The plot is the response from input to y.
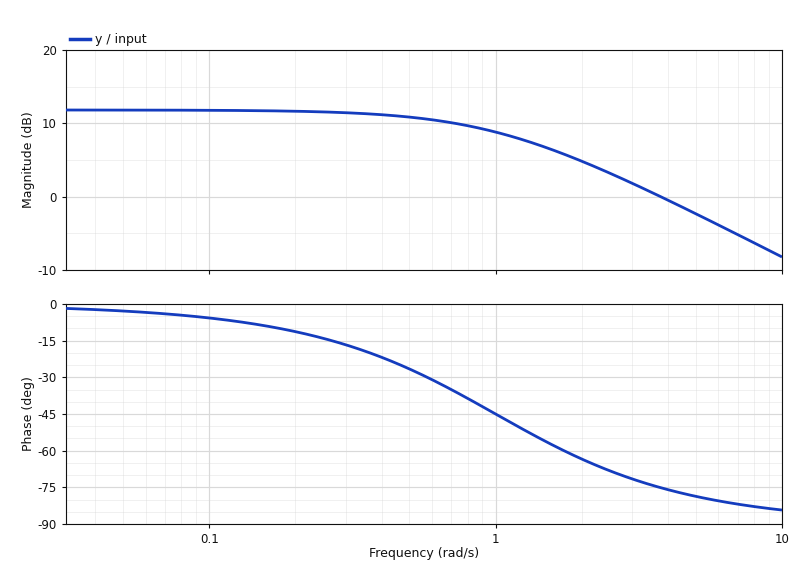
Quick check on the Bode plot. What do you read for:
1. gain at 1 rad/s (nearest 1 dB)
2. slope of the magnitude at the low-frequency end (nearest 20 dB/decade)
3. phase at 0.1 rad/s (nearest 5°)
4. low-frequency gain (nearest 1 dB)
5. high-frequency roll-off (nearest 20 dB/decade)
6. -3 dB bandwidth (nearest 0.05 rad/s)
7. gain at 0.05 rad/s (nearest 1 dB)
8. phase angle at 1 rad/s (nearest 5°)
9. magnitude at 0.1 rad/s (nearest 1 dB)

9 dB
0 dB/decade
-5°
12 dB
-20 dB/decade
1.00 rad/s
12 dB
-45°
12 dB
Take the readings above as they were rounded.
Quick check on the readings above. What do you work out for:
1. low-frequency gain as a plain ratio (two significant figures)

4.0
